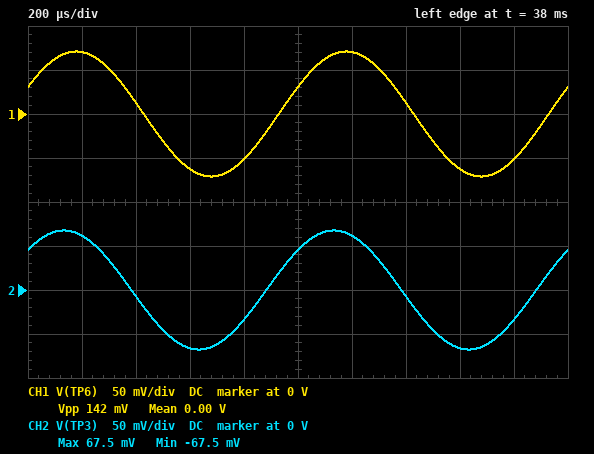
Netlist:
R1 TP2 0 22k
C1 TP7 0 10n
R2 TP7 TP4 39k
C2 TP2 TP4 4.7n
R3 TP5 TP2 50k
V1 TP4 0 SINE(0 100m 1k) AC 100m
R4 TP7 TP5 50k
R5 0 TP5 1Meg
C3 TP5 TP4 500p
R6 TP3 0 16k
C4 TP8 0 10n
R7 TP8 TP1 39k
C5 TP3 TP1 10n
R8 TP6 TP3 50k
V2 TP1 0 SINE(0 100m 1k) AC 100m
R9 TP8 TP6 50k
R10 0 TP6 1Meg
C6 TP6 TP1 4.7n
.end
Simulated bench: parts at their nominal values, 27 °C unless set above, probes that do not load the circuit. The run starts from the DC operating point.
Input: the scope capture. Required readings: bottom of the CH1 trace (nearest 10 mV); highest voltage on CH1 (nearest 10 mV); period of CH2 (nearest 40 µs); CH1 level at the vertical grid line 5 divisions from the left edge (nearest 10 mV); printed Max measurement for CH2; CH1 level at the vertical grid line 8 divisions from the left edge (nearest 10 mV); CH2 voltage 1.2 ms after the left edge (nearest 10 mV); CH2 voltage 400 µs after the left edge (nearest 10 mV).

-70 mV
70 mV
1.00 ms
30 mV
67.5 mV
-60 mV
60 mV
-10 mV
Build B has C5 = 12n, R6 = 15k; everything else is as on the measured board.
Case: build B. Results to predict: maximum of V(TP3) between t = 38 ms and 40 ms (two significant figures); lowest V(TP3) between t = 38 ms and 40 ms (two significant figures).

72 mV
-72 mV
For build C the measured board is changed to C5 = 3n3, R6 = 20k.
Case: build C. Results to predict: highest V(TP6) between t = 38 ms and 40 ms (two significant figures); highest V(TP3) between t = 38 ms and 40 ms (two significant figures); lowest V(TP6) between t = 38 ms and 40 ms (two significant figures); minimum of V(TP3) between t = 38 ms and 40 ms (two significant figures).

63 mV
40 mV
-63 mV
-40 mV
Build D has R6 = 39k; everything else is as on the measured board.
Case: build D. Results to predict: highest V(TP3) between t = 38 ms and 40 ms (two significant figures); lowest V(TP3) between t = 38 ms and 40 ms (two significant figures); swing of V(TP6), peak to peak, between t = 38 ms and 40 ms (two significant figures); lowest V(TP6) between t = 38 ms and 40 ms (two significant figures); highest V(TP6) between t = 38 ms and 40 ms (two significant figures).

88 mV
-88 mV
150 mV
-73 mV
73 mV
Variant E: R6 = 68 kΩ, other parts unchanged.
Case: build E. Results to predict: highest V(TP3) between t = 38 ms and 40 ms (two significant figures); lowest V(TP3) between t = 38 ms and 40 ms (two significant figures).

94 mV
-94 mV
